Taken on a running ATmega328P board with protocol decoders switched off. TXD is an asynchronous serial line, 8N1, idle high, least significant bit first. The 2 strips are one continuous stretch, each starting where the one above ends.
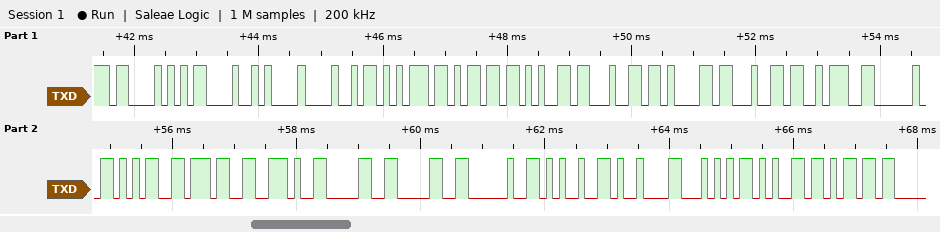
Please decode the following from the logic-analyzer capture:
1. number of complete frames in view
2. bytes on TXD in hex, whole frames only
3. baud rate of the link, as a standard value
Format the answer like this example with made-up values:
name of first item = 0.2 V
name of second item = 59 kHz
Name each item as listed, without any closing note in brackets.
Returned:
number of complete frames in view = 23
bytes on TXD in hex, whole frames only = 43 0D 0A 48 75 6D 65 64 61 64 3A 20 35 37 2E 30 30 20 25 09 54 65 6D
baud rate of the link, as a standard value = 9600 baud
